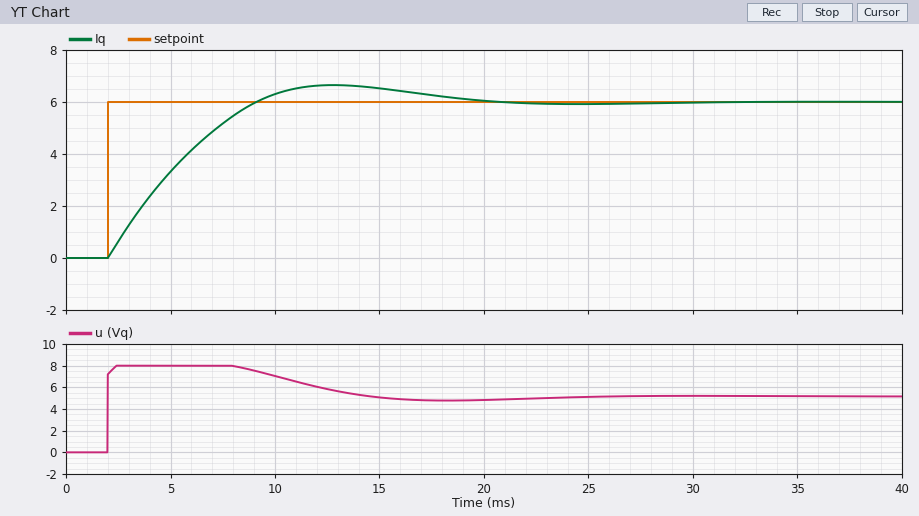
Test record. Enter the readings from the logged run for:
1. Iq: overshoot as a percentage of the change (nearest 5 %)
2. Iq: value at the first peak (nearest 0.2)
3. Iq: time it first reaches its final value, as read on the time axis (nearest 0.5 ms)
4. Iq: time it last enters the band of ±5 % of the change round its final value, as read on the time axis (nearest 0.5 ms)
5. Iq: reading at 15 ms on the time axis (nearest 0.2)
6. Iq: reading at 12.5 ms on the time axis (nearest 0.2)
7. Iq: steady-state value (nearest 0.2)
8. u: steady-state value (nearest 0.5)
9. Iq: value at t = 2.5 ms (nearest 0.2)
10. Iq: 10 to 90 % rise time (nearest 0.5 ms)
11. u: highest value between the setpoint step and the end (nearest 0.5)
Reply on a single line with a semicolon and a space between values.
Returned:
10 %; 6.6; 9.0 ms; 17.0 ms; 6.6; 6.6; 6.0; 5.0; 0.6; 5.5 ms; 8.0
